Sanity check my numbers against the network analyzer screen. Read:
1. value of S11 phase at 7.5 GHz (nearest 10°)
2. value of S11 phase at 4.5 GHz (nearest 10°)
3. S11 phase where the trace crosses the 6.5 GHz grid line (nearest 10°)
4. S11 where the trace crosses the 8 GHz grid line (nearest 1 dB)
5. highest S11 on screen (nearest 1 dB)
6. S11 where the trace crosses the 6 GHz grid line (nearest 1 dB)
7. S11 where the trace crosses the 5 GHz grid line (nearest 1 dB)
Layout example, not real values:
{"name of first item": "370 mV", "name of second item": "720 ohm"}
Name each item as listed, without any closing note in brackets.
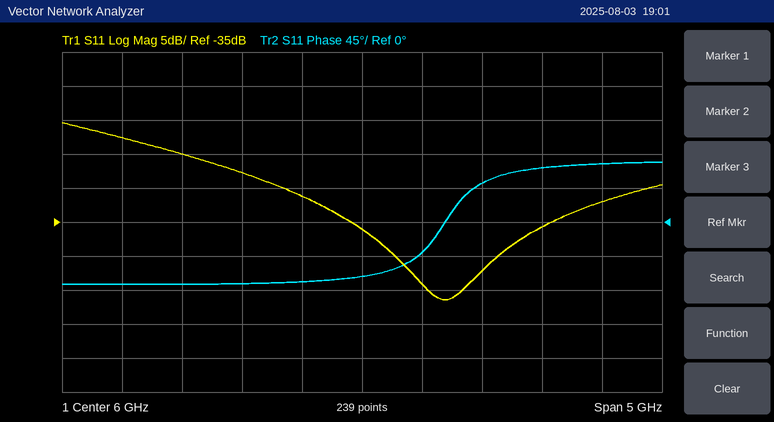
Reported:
{"value of S11 phase at 7.5 GHz": "70°", "value of S11 phase at 4.5 GHz": "-80°", "S11 phase where the trace crosses the 6.5 GHz grid line": "-40°", "S11 where the trace crosses the 8 GHz grid line": "-32 dB", "highest S11 on screen": "-20 dB", "S11 where the trace crosses the 6 GHz grid line": "-36 dB", "S11 where the trace crosses the 5 GHz grid line": "-28 dB"}
